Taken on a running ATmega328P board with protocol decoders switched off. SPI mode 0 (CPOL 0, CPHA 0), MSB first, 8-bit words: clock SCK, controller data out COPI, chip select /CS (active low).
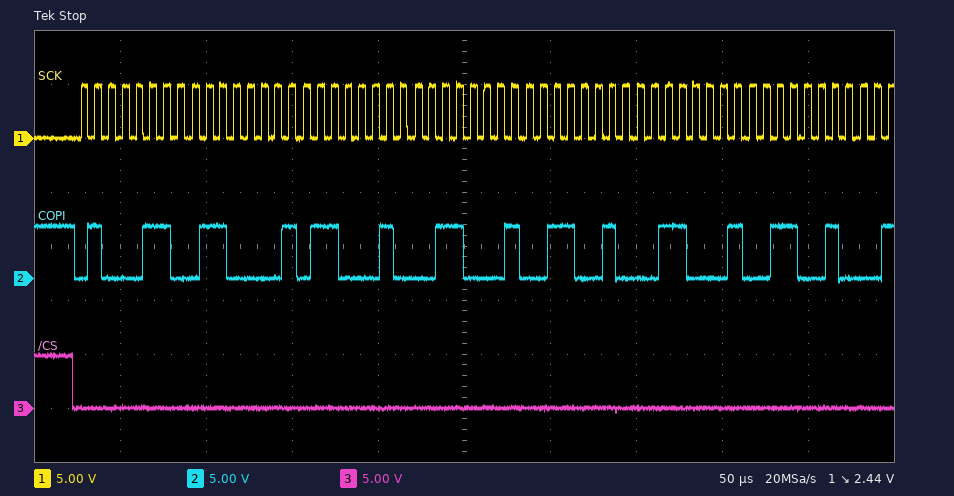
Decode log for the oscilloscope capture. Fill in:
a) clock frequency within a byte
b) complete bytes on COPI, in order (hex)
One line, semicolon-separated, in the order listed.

125 kHz; 46 61 62 31 32 31 32
